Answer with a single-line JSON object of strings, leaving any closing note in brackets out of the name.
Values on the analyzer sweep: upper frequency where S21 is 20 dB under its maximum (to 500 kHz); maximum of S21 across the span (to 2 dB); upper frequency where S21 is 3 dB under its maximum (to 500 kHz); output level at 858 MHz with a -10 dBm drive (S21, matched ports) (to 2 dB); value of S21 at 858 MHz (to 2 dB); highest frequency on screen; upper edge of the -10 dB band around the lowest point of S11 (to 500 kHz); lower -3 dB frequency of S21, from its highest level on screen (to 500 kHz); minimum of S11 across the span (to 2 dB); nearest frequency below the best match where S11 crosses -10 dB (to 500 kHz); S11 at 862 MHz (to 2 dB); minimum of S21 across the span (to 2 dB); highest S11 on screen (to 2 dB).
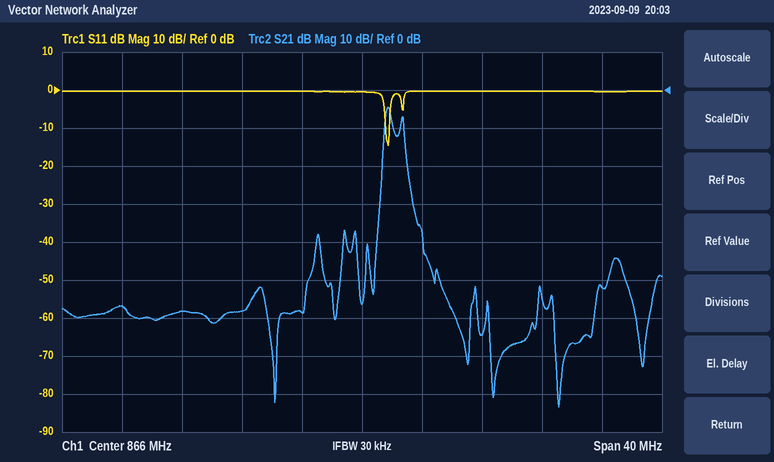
{"upper frequency where S21 is 20 dB under its maximum": "869.0 MHz", "maximum of S21 across the span": "-4 dB", "upper frequency where S21 is 3 dB under its maximum": "868.0 MHz", "output level at 858 MHz with a -10 dBm drive (S21, matched ports)": "-68 dBm", "value of S21 at 858 MHz": "-58 dB", "highest frequency on screen": "886 MHz", "upper edge of the -10 dB band around the lowest point of S11": "868.0 MHz", "lower -3 dB frequency of S21, from its highest level on screen": "867.5 MHz", "minimum of S11 across the span": "-14 dB", "nearest frequency below the best match where S11 crosses -10 dB": "867.5 MHz", "S11 at 862 MHz": "0 dB", "minimum of S21 across the span": "-84 dB", "highest S11 on screen": "0 dB"}
